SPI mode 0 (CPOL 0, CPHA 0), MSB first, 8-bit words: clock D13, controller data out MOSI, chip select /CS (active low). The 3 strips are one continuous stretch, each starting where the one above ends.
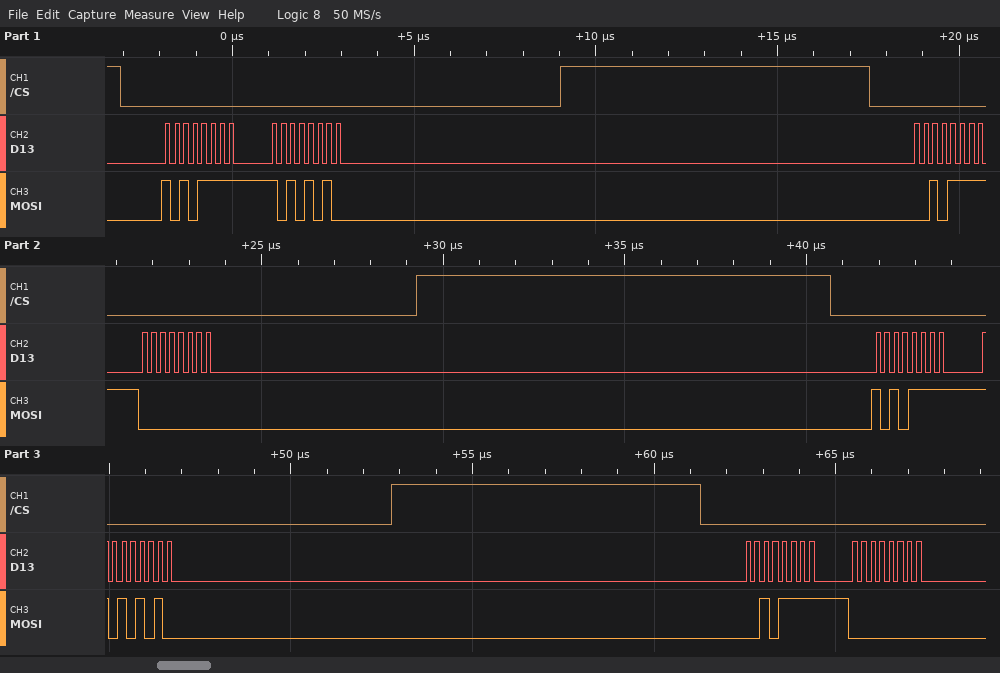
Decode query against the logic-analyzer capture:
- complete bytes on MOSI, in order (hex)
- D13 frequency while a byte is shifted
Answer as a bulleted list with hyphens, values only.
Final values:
- AF AA 2F 00 AF AA 2F 00
- 4 MHz
